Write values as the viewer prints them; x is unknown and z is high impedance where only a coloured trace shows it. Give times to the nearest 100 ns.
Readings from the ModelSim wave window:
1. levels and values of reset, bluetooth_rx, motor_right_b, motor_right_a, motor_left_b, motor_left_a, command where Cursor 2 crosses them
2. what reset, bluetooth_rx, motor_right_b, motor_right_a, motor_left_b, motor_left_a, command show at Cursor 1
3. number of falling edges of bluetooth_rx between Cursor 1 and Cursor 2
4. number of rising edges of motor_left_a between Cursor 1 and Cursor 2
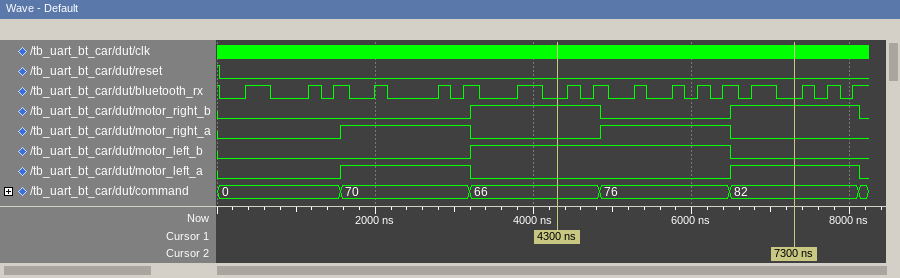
reset=0, bluetooth_rx=0, motor_right_b=1, motor_right_a=0, motor_left_b=0, motor_left_a=1, command=82
reset=0, bluetooth_rx=0, motor_right_b=1, motor_right_a=0, motor_left_b=1, motor_left_a=0, command=66
7
1
